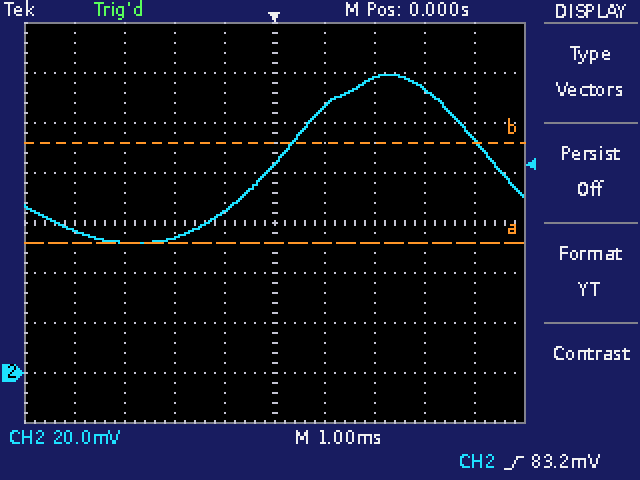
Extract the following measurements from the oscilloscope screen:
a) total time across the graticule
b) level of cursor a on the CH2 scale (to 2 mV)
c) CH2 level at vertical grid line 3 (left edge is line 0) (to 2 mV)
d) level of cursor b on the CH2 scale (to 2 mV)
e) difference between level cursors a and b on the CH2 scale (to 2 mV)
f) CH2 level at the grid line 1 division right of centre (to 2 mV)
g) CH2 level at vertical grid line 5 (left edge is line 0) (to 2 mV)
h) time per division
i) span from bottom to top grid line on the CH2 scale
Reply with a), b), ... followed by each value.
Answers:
a) 10 ms
b) 52 mV
c) 54 mV
d) 92 mV
e) 40 mV
f) 106 mV
g) 84 mV
h) 1 ms
i) 160 mV
